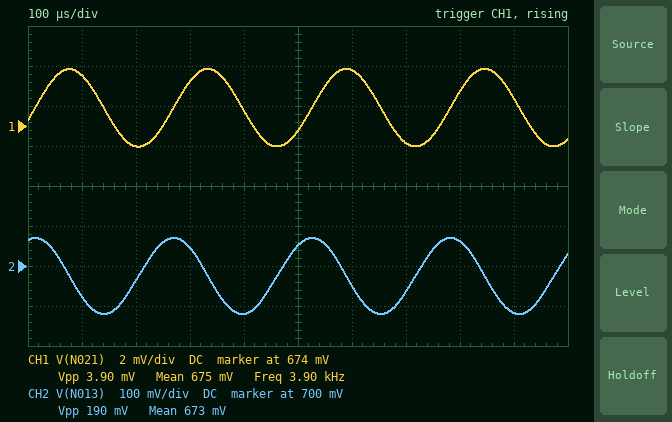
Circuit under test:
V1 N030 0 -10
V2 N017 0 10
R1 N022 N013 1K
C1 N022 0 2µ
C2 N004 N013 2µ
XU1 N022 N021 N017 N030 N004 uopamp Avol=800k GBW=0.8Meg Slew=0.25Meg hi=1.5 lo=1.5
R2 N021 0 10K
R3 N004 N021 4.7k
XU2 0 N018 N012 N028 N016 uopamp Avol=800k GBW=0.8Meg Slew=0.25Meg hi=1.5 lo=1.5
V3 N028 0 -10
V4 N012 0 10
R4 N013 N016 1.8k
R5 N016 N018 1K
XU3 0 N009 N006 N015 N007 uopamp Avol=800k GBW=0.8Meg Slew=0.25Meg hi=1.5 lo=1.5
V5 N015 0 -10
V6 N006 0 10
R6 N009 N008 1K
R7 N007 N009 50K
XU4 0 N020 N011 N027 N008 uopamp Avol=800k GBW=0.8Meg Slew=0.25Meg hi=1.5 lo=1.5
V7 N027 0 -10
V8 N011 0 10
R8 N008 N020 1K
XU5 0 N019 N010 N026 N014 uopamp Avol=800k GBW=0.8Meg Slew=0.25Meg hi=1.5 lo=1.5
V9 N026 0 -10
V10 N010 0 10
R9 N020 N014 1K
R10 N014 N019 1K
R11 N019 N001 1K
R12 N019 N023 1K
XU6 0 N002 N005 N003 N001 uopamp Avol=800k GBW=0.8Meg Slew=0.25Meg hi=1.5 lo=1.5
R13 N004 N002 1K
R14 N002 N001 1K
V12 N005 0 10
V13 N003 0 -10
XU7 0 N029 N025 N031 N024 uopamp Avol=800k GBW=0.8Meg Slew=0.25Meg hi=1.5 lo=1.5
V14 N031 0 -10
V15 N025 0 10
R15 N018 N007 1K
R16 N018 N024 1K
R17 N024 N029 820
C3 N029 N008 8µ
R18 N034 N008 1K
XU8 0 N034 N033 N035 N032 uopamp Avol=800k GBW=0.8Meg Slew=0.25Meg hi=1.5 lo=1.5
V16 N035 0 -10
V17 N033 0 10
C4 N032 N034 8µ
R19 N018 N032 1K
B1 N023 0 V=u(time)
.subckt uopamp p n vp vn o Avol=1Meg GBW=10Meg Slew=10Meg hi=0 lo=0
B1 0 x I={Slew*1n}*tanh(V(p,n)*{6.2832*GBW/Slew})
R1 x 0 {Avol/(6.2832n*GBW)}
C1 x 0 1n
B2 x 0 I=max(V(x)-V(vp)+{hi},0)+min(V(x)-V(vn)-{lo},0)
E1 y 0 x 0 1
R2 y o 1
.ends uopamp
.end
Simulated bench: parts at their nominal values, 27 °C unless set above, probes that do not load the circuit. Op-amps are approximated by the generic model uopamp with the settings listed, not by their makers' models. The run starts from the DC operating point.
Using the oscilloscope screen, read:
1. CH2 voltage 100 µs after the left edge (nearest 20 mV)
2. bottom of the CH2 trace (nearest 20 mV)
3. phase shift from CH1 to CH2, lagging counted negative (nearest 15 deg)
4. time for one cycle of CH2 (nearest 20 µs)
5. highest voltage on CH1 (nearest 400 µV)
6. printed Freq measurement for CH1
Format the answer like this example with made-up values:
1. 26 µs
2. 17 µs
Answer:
1. 620 mV
2. 580 mV
3. 90 deg
4. 260 µs
5. 676.8 mV
6. 3.90 kHz
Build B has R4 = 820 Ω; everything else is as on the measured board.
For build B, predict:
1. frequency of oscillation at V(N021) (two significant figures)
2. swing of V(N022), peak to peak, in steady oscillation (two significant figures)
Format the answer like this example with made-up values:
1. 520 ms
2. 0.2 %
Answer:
1. 3.8 kHz
2. 9.3 mV
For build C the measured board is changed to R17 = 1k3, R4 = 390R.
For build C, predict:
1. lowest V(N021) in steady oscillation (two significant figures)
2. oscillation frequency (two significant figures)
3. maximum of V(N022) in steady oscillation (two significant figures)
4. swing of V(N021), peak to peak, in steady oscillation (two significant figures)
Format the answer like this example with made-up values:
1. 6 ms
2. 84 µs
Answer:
1. 640 mV
2. 2.6 kHz
3. 690 mV
4. 47 mV
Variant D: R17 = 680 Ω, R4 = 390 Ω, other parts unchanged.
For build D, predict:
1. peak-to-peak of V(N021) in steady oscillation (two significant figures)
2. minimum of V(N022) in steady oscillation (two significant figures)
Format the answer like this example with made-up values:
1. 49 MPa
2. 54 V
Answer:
1. 19 mV
2. 660 mV
